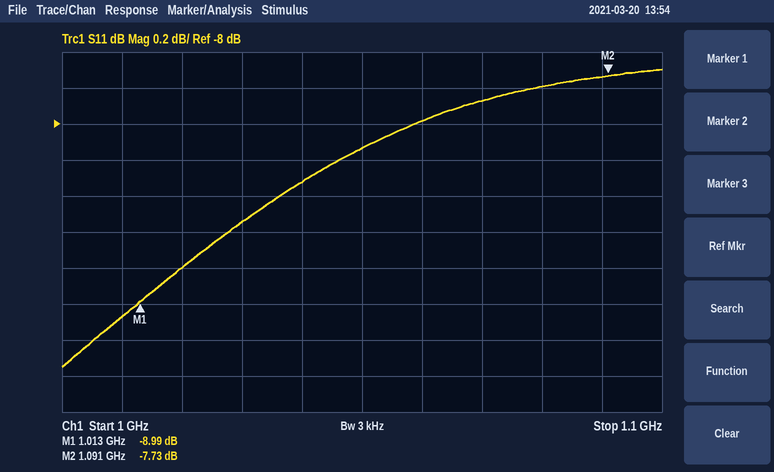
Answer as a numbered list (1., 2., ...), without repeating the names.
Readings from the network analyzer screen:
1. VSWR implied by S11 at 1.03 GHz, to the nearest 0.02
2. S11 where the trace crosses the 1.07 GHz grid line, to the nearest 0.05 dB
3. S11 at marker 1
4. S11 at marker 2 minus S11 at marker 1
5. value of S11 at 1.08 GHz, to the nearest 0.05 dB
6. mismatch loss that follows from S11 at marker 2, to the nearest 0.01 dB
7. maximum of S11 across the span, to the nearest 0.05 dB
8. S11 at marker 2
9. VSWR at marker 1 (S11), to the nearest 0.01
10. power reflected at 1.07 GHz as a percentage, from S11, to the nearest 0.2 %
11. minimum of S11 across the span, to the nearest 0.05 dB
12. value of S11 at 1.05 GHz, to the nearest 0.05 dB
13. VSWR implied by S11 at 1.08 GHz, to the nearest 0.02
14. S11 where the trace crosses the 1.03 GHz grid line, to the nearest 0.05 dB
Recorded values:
1. 2.20
2. -7.85 dB
3. -8.99 dB
4. 1.26 dB
5. -7.80 dB
6. 0.80 dB
7. -7.70 dB
8. -7.73 dB
9. 2.10
10. 16.4 %
11. -9.35 dB
12. -8.15 dB
13. 2.38
14. -8.55 dB
